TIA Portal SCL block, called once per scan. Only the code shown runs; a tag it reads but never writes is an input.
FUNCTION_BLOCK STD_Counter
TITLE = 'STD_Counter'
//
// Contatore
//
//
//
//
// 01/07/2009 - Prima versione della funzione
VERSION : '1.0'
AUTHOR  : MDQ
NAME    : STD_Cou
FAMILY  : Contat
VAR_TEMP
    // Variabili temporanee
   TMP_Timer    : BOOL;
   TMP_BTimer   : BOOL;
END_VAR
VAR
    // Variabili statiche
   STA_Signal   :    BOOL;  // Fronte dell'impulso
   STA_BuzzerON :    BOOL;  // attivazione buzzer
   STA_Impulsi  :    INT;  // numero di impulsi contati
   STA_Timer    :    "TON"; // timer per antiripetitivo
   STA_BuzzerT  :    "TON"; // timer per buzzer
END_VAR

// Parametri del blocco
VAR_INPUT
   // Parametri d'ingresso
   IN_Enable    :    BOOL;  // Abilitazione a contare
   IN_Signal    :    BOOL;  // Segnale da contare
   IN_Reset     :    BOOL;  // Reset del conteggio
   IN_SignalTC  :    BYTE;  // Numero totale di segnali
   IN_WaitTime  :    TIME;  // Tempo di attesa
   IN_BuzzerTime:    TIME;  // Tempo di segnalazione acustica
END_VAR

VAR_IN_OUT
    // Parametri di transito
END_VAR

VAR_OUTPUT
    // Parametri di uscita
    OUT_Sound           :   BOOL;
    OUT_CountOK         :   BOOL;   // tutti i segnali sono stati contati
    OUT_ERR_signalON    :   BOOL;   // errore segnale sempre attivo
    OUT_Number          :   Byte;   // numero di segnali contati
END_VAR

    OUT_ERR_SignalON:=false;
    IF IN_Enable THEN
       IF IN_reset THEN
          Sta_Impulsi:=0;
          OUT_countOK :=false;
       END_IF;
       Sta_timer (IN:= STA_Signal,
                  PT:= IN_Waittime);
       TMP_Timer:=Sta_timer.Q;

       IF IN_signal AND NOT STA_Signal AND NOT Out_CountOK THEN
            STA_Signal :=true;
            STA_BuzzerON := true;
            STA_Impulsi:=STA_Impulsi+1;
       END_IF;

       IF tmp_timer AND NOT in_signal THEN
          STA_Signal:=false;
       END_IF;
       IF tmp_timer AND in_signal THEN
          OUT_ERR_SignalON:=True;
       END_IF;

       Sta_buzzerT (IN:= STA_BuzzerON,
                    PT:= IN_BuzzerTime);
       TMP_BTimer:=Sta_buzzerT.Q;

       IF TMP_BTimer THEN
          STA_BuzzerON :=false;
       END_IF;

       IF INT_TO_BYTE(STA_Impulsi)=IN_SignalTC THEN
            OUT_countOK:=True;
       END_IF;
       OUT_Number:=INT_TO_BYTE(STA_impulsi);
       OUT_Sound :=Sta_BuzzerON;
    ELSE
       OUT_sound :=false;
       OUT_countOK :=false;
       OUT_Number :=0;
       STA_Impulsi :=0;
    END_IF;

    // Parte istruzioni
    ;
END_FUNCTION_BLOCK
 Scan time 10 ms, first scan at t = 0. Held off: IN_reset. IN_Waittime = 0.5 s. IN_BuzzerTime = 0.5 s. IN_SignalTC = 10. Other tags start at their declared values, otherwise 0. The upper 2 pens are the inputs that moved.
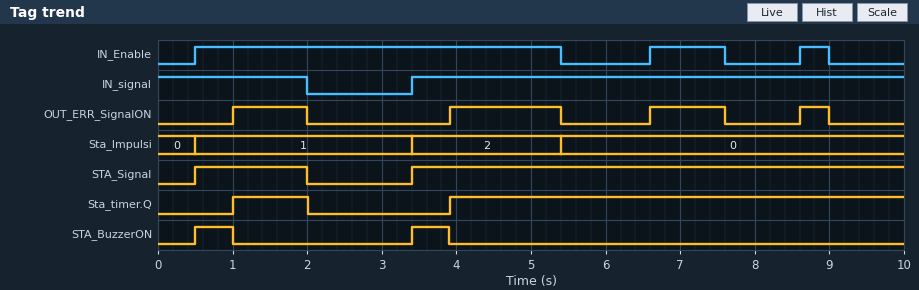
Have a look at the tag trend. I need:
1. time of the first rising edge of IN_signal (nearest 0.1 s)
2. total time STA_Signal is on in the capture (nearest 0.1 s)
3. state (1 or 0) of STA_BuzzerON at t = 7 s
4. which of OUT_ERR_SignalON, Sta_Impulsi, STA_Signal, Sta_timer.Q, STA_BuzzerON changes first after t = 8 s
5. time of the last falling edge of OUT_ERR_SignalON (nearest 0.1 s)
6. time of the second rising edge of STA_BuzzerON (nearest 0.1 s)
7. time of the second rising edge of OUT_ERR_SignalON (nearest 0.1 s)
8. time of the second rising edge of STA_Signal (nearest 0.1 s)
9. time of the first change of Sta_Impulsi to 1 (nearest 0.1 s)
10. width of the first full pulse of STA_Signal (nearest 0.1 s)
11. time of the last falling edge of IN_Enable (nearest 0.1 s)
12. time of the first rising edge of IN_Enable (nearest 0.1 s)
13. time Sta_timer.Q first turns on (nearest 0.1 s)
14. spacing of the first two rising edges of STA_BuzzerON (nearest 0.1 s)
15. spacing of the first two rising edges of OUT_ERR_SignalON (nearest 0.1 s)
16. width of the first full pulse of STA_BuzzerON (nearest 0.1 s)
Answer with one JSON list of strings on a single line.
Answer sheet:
["3.4 s", "8.1 s", "0", "OUT_ERR_SignalON", "9.0 s", "3.4 s", "3.9 s", "3.4 s", "0.5 s", "1.5 s", "9.0 s", "0.5 s", "1.0 s", "2.9 s", "2.9 s", "0.5 s"]
